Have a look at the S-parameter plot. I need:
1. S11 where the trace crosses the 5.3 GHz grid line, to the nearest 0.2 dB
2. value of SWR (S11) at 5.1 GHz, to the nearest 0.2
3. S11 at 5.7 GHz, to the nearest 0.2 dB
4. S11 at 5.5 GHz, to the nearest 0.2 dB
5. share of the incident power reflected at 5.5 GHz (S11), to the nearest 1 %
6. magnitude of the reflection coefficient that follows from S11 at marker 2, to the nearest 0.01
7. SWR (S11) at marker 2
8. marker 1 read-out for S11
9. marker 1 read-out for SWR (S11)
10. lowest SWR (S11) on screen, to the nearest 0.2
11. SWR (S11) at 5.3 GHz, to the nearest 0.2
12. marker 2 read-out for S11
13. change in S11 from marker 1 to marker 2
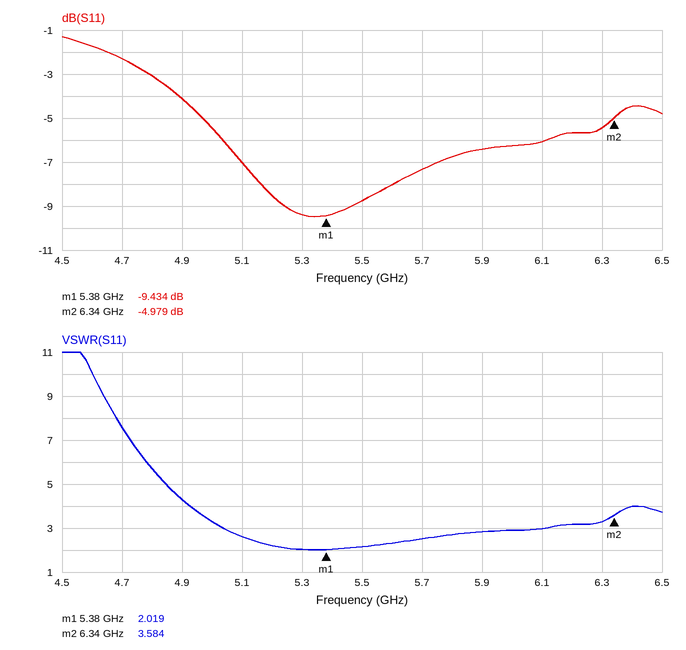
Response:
-9.4 dB
2.6
-7.4 dB
-8.8 dB
13 %
0.56
3.584
-9.434 dB
2.019
2.0
2.0
-4.979 dB
4.455 dB
